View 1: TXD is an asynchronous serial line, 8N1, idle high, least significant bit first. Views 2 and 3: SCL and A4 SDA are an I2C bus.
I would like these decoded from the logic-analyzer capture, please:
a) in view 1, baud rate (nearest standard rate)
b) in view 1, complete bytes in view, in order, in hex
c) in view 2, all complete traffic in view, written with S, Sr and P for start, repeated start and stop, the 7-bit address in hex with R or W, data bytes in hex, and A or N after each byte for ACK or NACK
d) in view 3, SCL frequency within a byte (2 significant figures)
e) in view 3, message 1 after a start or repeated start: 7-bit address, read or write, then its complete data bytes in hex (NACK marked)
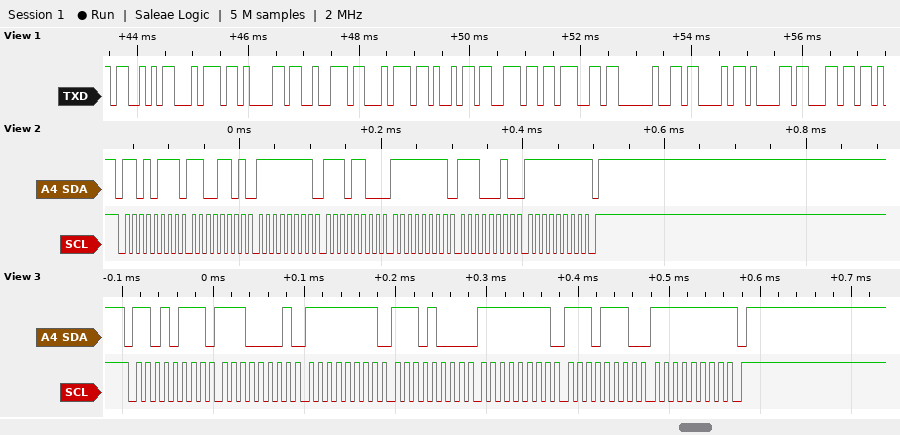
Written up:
9600 baud
53 74 61 72 74 69 6E 67 20 43 61 6C
S 6BR A CD A FF A EC A FF A E2 A FF N P
100 kHz
0x6B read: E1 FF E8 FF EE FF NACK
